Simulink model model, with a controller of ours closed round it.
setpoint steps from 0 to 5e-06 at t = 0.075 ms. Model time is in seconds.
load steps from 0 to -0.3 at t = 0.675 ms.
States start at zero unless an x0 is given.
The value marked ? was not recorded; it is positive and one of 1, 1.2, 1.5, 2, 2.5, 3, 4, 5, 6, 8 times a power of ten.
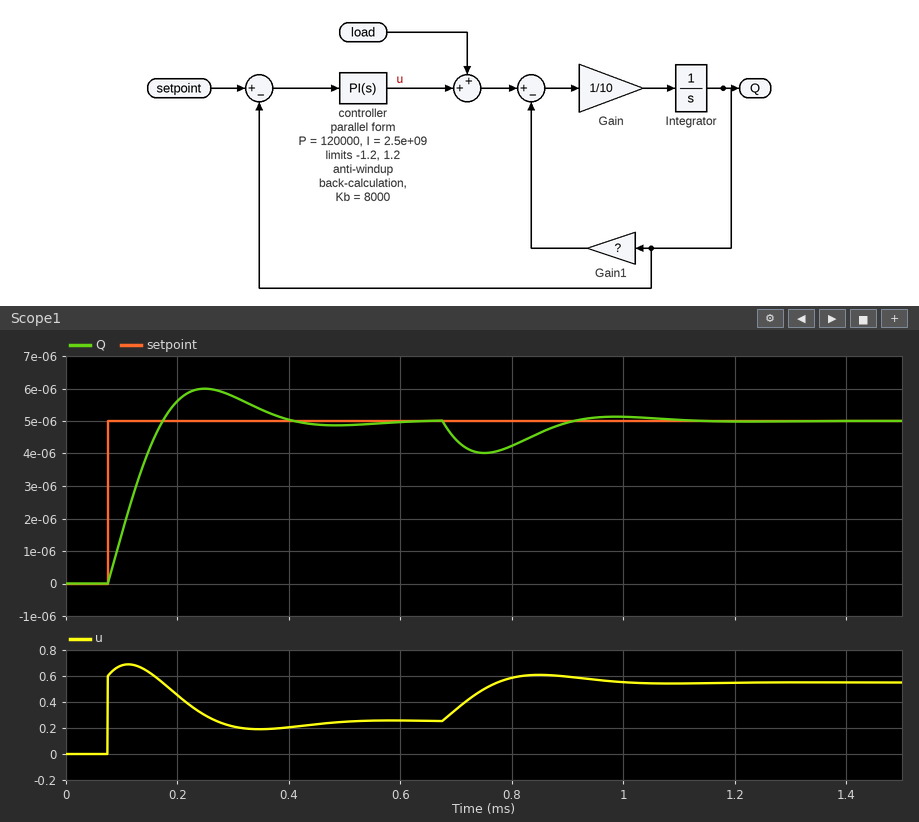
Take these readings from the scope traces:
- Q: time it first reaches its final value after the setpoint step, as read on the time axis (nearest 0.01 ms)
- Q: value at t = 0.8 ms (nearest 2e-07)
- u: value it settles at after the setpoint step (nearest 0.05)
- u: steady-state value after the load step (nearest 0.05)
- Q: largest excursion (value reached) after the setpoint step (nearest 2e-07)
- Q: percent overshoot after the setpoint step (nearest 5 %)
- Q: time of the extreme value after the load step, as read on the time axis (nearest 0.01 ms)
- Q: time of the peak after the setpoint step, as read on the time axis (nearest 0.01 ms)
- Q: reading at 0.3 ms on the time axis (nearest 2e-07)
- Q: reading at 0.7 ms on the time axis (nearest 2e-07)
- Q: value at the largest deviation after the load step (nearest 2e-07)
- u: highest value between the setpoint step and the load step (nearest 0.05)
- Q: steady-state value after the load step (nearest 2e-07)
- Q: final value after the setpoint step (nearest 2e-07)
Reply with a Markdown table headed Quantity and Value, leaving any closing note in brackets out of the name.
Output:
| Quantity | Value |
|---|---|
| Q: time it first reaches its final value after the setpoint step, as read on the time axis | 0.17 ms |
| Q: value at t = 0.8 ms | 0.0000042 |
| u: value it settles at after the setpoint step | 0.25 |
| u: steady-state value after the load step | 0.55 |
| Q: largest excursion (value reached) after the setpoint step | 0.0000060 |
| Q: percent overshoot after the setpoint step | 20 % |
| Q: time of the extreme value after the load step, as read on the time axis | 0.75 ms |
| Q: time of the peak after the setpoint step, as read on the time axis | 0.25 ms |
| Q: reading at 0.3 ms on the time axis | 0.0000058 |
| Q: reading at 0.7 ms on the time axis | 0.0000044 |
| Q: value at the largest deviation after the load step | 0.0000040 |
| u: highest value between the setpoint step and the load step | 0.70 |
| Q: steady-state value after the load step | 0.0000050 |
| Q: final value after the setpoint step | 0.0000050 |
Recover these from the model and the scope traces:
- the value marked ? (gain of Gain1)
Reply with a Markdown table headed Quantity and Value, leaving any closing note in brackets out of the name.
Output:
| Quantity | Value |
|---|---|
| the value marked ? | 50000 |
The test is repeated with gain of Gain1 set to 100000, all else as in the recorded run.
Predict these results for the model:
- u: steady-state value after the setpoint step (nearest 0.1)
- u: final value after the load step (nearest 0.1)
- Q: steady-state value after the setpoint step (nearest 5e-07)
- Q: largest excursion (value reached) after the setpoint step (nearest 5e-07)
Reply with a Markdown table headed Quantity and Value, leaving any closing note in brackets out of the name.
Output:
| Quantity | Value |
|---|---|
| u: steady-state value after the setpoint step | 0.5 |
| u: final value after the load step | 0.8 |
| Q: steady-state value after the setpoint step | 0.0000050 |
| Q: largest excursion (value reached) after the setpoint step | 0.0000055 |
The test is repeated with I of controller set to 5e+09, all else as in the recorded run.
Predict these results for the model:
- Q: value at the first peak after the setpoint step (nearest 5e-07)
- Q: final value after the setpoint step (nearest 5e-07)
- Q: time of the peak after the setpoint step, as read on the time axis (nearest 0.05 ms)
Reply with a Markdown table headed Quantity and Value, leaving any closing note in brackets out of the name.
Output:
| Quantity | Value |
|---|---|
| Q: value at the first peak after the setpoint step | 0.0000065 |
| Q: final value after the setpoint step | 0.0000050 |
| Q: time of the peak after the setpoint step, as read on the time axis | 0.20 ms |
